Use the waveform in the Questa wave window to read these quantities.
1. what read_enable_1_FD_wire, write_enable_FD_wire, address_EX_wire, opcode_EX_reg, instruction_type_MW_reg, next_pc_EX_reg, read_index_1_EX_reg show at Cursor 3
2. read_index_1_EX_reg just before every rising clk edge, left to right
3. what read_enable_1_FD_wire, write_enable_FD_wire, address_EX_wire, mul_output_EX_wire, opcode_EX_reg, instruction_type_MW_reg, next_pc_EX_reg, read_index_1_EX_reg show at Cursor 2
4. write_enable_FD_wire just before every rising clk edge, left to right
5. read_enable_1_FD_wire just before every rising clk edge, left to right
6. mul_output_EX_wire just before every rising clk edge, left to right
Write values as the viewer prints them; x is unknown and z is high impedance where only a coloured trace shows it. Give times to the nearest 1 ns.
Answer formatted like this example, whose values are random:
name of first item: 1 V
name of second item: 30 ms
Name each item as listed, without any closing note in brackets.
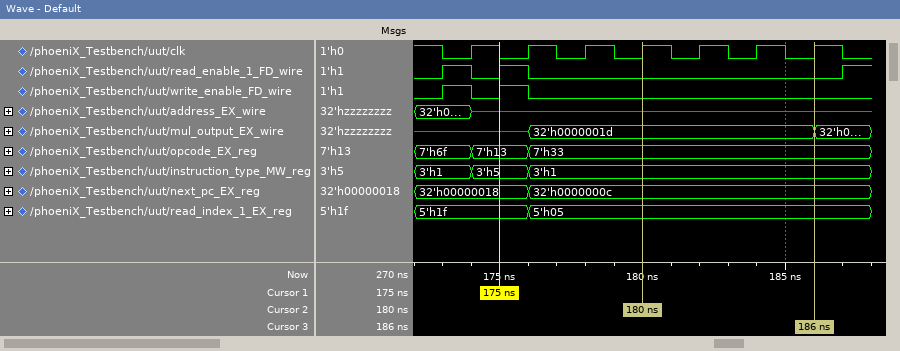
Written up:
what read_enable_1_FD_wire, write_enable_FD_wire, address_EX_wire, opcode_EX_reg, instruction_type_MW_reg, next_pc_EX_reg, read_index_1_EX_reg show at Cursor 3: read_enable_1_FD_wire=0, write_enable_FD_wire=0, address_EX_wire=z, opcode_EX_reg=7'h33, instruction_type_MW_reg=3'h1, next_pc_EX_reg=32'h0000000c, read_index_1_EX_reg=5'h05
read_index_1_EX_reg just before every rising clk edge, left to right: 5'h1f, 5'h1f, 5'h05, 5'h05, 5'h05, 5'h05, 5'h05
what read_enable_1_FD_wire, write_enable_FD_wire, address_EX_wire, mul_output_EX_wire, opcode_EX_reg, instruction_type_MW_reg, next_pc_EX_reg, read_index_1_EX_reg show at Cursor 2: read_enable_1_FD_wire=0, write_enable_FD_wire=0, address_EX_wire=z, mul_output_EX_wire=32'h0000001d, opcode_EX_reg=7'h33, instruction_type_MW_reg=3'h1, next_pc_EX_reg=32'h0000000c, read_index_1_EX_reg=5'h05
write_enable_FD_wire just before every rising clk edge, left to right: 1 1 0 0 0 0 0
read_enable_1_FD_wire just before every rising clk edge, left to right: 1 1 0 0 0 0 0
mul_output_EX_wire just before every rising clk edge, left to right: z, z, 32'h0000001d, 32'h0000001d, 32'h0000001d, 32'h0000001d, 32'h0000001d
